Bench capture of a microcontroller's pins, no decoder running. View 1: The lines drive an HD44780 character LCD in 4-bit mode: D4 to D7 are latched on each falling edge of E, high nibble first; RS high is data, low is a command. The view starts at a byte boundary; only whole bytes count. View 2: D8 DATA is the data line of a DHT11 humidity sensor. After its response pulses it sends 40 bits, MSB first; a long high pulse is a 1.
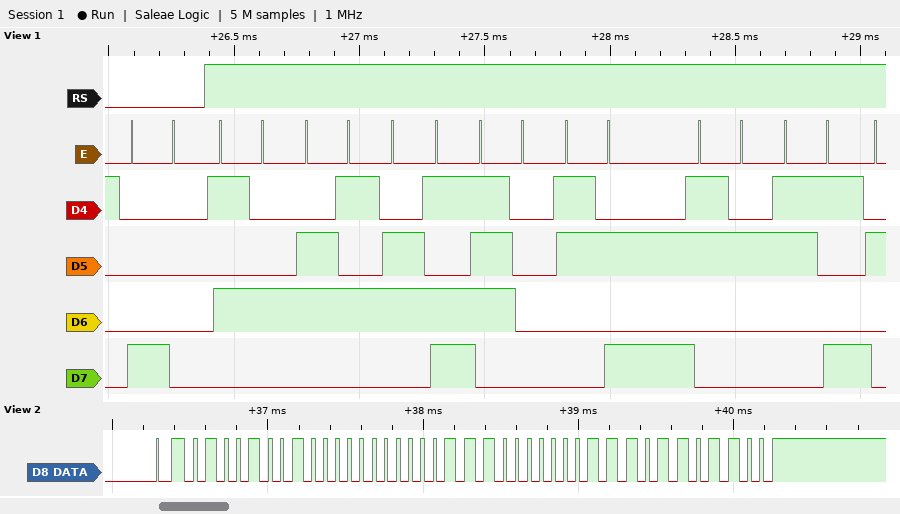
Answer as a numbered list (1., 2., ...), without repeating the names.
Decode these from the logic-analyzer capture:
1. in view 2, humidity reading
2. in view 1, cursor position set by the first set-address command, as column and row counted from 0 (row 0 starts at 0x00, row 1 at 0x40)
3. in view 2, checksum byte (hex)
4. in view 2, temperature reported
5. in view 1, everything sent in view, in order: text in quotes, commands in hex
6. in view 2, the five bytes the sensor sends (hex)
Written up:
1. 73 %
2. column 0, row 0
3. 0x6C
4. 28.7 °C
5. 0x80 "Temp:29"
6. 49 00 1C 07 6C
